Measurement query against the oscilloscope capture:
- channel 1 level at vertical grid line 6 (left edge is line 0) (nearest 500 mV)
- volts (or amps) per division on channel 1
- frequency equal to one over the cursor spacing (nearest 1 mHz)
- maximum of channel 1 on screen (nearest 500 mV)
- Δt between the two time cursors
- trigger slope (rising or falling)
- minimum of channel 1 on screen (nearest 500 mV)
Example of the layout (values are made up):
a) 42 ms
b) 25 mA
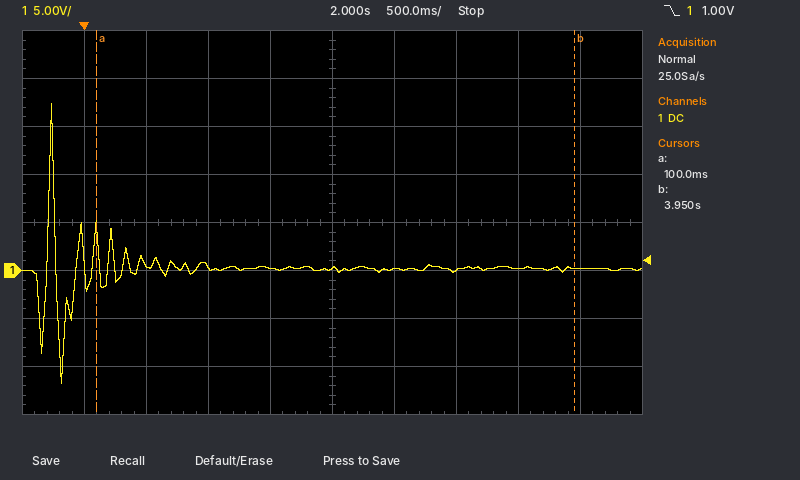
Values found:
a) 0.0 V
b) 5 V
c) 260 mHz
d) 17.5 V
e) 3.85 s
f) falling
g) -12.0 V
